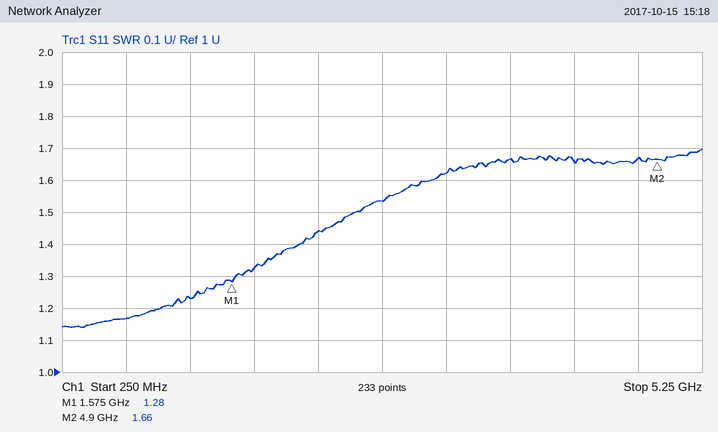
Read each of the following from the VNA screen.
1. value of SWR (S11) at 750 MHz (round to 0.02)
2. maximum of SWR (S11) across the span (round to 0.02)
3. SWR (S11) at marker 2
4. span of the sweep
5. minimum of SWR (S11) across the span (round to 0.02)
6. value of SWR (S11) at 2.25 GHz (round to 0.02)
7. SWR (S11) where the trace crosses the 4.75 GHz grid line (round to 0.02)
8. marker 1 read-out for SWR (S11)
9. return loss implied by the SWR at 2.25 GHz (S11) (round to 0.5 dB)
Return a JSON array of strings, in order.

["1.16", "1.70", "1.66", "5 GHz", "1.14", "1.44", "1.66", "1.28", "15.0 dB"]
